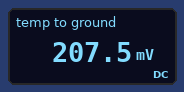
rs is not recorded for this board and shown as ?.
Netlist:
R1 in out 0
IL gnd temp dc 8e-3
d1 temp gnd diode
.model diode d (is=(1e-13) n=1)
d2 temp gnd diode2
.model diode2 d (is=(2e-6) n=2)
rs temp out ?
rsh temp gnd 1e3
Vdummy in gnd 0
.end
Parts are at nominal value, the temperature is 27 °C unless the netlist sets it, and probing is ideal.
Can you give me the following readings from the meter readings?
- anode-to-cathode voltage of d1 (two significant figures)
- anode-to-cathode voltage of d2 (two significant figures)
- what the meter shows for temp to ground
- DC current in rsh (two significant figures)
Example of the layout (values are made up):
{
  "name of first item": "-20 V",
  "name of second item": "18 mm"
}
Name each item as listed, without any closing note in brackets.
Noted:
{
  "anode-to-cathode voltage of d1": "210 mV",
  "anode-to-cathode voltage of d2": "210 mV",
  "what the meter shows for temp to ground": "207.5 mV",
  "DC current in rsh": "210 µA"
}
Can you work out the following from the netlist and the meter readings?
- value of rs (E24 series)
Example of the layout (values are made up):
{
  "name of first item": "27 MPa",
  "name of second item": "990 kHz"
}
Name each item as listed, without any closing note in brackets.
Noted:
{
  "value of rs": "27 Ω"
}
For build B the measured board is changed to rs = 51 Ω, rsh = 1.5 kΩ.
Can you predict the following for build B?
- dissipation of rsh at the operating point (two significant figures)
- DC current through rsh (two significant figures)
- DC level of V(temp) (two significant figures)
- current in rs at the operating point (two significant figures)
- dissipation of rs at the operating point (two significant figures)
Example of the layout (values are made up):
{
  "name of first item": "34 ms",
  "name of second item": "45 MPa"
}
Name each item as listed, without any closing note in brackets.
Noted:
{
  "dissipation of rsh at the operating point": "74 µW",
  "DC current through rsh": "220 µA",
  "DC level of V(temp)": "330 mV",
  "current in rs at the operating point": "6.5 mA",
  "dissipation of rs at the operating point": "2.2 mW"
}
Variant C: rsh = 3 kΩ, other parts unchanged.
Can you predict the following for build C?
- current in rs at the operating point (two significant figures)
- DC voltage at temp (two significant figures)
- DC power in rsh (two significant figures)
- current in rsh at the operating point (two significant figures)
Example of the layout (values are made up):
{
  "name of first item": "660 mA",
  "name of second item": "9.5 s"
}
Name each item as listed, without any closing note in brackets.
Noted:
{
  "current in rs at the operating point": "7.8 mA",
  "DC voltage at temp": "210 mV",
  "DC power in rsh": "15 µW",
  "current in rsh at the operating point": "70 µA"
}
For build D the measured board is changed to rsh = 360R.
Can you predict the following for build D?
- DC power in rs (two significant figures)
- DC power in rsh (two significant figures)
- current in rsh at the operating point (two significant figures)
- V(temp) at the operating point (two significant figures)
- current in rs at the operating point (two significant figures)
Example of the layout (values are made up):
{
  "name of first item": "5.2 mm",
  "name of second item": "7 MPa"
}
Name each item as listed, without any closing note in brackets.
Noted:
{
  "DC power in rs": "1.5 mW",
  "DC power in rsh": "110 µW",
  "current in rsh at the operating point": "550 µA",
  "V(temp) at the operating point": "200 mV",
  "current in rs at the operating point": "7.4 mA"
}
